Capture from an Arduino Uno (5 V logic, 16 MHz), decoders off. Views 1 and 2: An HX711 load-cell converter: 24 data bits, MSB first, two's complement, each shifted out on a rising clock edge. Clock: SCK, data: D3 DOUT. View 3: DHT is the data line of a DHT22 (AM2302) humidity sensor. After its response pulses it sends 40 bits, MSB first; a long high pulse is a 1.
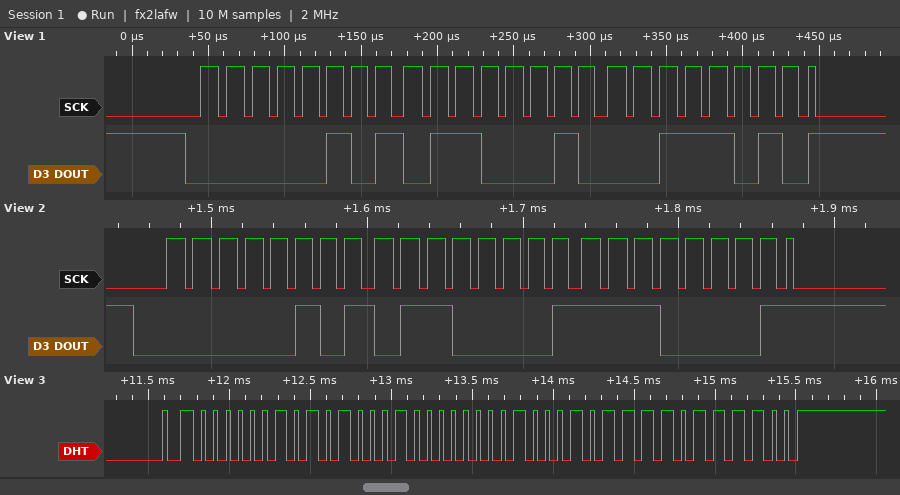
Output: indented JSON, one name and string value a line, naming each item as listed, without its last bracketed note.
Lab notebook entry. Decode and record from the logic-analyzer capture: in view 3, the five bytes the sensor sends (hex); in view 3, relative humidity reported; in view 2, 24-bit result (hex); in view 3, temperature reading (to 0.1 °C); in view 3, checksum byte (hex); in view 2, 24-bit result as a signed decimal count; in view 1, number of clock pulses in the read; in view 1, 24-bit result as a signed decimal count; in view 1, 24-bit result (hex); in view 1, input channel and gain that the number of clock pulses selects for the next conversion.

{
  "in view 3, the five bytes the sensor sends": "02 A2 01 17 BC",
  "in view 3, relative humidity reported": "67.4 %",
  "in view 2, 24-bit result": "0x0561E1",
  "in view 3, temperature reading": "27.9 °C",
  "in view 3, checksum byte": "0xBC",
  "in view 2, 24-bit result as a signed decimal count": "352737",
  "in view 1, number of clock pulses in the read": "25",
  "in view 1, 24-bit result as a signed decimal count": "352826",
  "in view 1, 24-bit result": "0x05623A",
  "in view 1, input channel and gain that the number of clock pulses selects for the next conversion": "channel A, gain 128"
}
